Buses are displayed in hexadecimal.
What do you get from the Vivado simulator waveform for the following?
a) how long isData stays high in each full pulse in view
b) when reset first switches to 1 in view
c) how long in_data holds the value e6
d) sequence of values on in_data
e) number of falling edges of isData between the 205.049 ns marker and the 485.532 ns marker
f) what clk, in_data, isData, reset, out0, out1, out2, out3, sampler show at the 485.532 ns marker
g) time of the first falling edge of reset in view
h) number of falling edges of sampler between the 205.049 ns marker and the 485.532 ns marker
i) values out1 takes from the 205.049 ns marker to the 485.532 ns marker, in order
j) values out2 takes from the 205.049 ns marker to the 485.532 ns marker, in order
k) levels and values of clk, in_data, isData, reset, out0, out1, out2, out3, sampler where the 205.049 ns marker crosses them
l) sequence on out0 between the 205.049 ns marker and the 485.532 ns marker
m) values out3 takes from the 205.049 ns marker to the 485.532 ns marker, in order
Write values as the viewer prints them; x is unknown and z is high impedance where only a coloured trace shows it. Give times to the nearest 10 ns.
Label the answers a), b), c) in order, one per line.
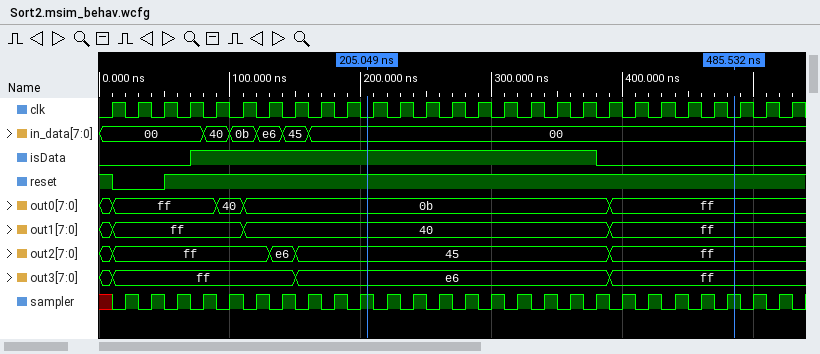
a) 310 ns
b) 50 ns
c) 20 ns
d) 00, 40, 0b, e6, 45, 00
e) 1
f) clk=0, in_data=00, isData=0, reset=1, out0=ff, out1=ff, out2=ff, out3=ff, sampler=1
g) 10 ns
h) 14
i) 40, ff
j) 45, ff
k) clk=0, in_data=00, isData=1, reset=1, out0=0b, out1=40, out2=45, out3=e6, sampler=1
l) 0b, ff
m) e6, ff
